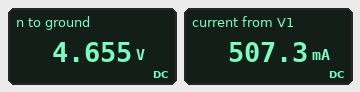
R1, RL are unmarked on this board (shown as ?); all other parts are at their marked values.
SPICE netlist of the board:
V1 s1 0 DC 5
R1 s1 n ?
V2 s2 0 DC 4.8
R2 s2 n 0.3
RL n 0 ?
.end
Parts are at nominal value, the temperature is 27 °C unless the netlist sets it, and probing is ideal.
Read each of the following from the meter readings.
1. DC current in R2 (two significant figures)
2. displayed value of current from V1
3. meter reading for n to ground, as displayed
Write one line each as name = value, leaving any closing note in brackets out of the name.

DC current in R2 = 480 mA
displayed value of current from V1 = 507.3 mA
meter reading for n to ground, as displayed = 4.655 V
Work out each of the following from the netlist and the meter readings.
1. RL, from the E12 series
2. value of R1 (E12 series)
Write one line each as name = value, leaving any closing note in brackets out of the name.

RL, from the E12 series = 4.7 Ω
value of R1 = 0.68 Ω
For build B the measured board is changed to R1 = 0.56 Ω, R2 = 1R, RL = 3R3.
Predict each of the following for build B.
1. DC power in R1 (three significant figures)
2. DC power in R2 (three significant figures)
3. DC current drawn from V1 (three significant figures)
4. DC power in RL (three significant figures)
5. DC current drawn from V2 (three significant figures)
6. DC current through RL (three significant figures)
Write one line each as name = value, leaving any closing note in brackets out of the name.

DC power in R1 = 551 mW
DC power in R2 = 126 mW
DC current drawn from V1 = 992 mA
DC power in RL = 5.99 W
DC current drawn from V2 = 355 mA
DC current through RL = 1.35 A
